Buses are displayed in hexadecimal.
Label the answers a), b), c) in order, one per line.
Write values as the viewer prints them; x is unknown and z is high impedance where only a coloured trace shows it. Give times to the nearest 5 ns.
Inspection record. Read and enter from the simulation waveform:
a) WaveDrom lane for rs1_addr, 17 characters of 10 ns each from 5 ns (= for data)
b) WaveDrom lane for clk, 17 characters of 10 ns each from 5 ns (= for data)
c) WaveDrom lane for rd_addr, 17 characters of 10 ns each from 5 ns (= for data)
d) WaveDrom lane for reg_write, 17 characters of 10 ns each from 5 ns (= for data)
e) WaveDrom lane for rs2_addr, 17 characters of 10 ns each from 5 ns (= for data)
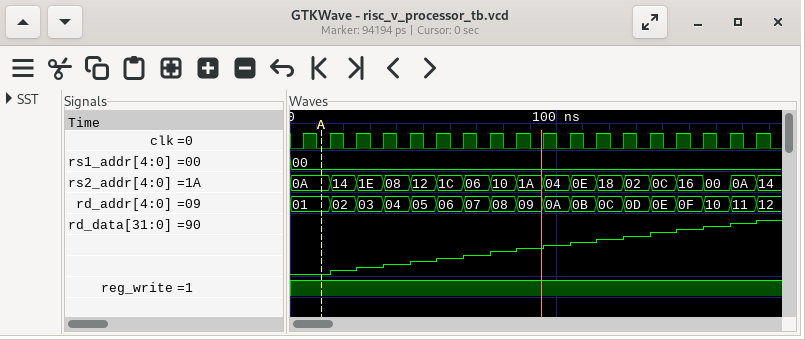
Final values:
a) {name: 'rs1_addr', wave: '=................', data: '00'}
b) {name: 'clk', wave: 'p................'}
c) {name: 'rd_addr', wave: '=================', data: '01 02 03 04 05 06 07 08 09 0A 0B 0C 0D 0E 0F 10 11'}
d) {name: 'reg_write', wave: '1................'}
e) {name: 'rs2_addr', wave: '=================', data: '0A 14 1E 08 12 1C 06 10 1A 04 0E 18 02 0C 16 00 0A'}
